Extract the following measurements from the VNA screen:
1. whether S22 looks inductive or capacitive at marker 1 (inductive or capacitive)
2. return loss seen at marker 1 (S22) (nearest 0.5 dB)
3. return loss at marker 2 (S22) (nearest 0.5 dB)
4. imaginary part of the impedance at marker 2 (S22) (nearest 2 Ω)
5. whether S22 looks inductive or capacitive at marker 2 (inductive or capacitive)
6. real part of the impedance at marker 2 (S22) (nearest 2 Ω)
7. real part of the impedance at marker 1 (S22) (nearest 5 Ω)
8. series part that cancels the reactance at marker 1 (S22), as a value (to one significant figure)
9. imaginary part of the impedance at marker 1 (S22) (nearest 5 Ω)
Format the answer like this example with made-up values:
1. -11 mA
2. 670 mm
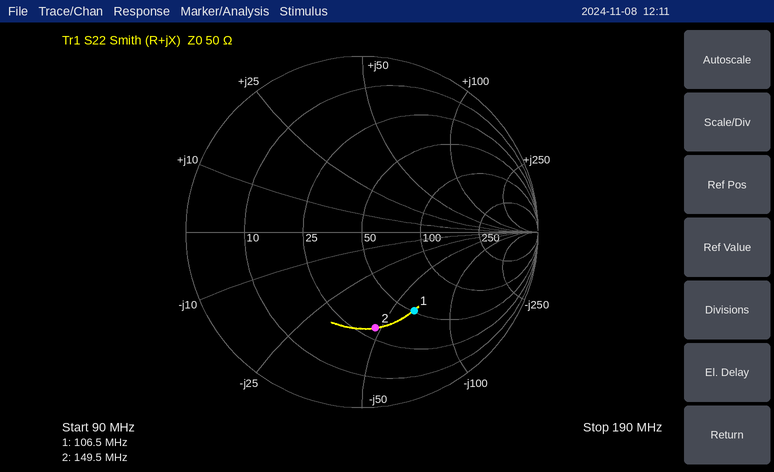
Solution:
1. capacitive
2. 5.5 dB
3. 5.0 dB
4. -48 Ω
5. capacitive
6. 30 Ω
7. 50 Ω
8. 100 nH
9. -65 Ω
